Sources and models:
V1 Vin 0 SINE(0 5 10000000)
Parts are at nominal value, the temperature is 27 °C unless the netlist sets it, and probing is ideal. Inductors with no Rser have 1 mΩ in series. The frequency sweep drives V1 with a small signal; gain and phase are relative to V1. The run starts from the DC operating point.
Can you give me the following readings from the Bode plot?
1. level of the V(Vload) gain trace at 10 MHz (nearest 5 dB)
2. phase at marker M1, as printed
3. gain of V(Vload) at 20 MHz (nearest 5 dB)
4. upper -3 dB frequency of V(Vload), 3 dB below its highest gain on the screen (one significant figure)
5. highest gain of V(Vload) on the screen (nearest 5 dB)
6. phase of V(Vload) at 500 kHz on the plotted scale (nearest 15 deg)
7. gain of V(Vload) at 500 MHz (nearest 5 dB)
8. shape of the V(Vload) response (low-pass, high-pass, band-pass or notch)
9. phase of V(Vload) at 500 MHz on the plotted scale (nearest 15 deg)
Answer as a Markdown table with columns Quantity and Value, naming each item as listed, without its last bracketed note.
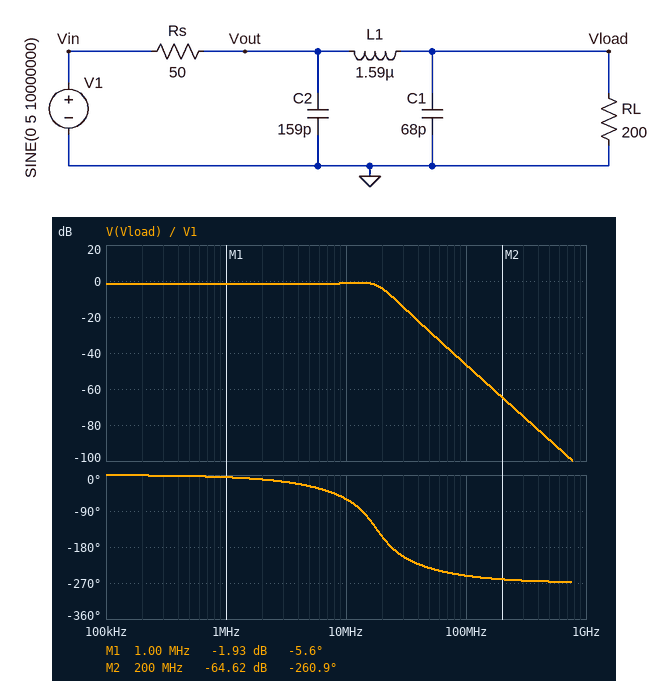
| Quantity | Value |
|---|---|
| level of the V(Vload) gain trace at 10 MHz | 0 dB |
| phase at marker M1, as printed | -5.6 deg |
| gain of V(Vload) at 20 MHz | -5 dB |
| upper -3 dB frequency of V(Vload), 3 dB below its highest gain on the screen | 20 MHz |
| highest gain of V(Vload) on the screen | 0 dB |
| phase of V(Vload) at 500 kHz on the plotted scale | 0 deg |
| gain of V(Vload) at 500 MHz | -90 dB |
| shape of the V(Vload) response | low-pass |
| phase of V(Vload) at 500 MHz on the plotted scale | -270 deg |
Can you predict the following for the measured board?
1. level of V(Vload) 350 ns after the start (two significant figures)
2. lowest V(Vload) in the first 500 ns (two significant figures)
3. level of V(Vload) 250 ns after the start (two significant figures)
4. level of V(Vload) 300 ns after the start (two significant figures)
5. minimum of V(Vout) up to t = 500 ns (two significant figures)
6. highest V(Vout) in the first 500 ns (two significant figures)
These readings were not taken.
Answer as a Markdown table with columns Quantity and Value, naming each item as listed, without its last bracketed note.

| Quantity | Value |
|---|---|
| level of V(Vload) 350 ns after the start | 3.8 V |
| lowest V(Vload) in the first 500 ns | -4.4 V |
| level of V(Vload) 250 ns after the start | 3.8 V |
| level of V(Vload) 300 ns after the start | -3.8 V |
| minimum of V(Vout) up to t = 500 ns | -3.3 V |
| highest V(Vout) in the first 500 ns | 3.6 V |
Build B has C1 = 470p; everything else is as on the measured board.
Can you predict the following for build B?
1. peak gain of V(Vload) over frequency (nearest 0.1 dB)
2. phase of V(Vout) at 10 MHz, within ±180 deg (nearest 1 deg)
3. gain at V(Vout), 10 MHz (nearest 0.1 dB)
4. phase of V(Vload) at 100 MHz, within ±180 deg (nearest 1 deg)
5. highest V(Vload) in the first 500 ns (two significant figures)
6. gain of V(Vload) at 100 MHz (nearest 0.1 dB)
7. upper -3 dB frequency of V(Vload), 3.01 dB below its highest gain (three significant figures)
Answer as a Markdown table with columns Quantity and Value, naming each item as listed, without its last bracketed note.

| Quantity | Value |
|---|---|
| peak gain of V(Vload) over frequency | -1.2 dB |
| phase of V(Vout) at 10 MHz, within ±180 deg | 13 deg |
| gain at V(Vout), 10 MHz | -0.7 dB |
| phase of V(Vload) at 100 MHz, within ±180 deg | 102 deg |
| highest V(Vload) in the first 500 ns | 2.6 V |
| gain of V(Vload) at 100 MHz | -63.4 dB |
| upper -3 dB frequency of V(Vload), 3.01 dB below its highest gain | 8.56 MHz |
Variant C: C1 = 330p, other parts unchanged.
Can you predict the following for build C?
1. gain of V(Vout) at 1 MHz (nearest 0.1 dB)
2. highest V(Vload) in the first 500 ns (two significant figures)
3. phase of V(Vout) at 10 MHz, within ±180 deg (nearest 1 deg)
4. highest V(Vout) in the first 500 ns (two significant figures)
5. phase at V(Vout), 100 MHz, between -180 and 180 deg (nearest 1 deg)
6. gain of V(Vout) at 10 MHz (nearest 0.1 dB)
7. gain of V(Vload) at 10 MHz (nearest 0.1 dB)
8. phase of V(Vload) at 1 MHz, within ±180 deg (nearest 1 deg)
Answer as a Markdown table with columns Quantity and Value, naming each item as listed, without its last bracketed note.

| Quantity | Value |
|---|---|
| gain of V(Vout) at 1 MHz | -2.1 dB |
| highest V(Vload) in the first 500 ns | 3.5 V |
| phase of V(Vout) at 10 MHz, within ±180 deg | 18 deg |
| highest V(Vout) in the first 500 ns | 4.0 V |
| phase at V(Vout), 100 MHz, between -180 and 180 deg | -79 deg |
| gain of V(Vout) at 10 MHz | -1.9 dB |
| gain of V(Vload) at 10 MHz | -3.3 dB |
| phase of V(Vload) at 1 MHz, within ±180 deg | -9 deg |
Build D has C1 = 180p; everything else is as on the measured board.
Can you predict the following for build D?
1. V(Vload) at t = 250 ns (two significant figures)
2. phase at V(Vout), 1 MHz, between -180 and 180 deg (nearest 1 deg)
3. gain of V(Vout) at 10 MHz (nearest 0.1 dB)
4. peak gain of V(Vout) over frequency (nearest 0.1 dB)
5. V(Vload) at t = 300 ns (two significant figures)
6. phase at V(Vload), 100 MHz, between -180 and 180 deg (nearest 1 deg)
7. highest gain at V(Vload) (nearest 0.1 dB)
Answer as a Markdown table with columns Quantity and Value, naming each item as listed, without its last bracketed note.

| Quantity | Value |
|---|---|
| V(Vload) at t = 250 ns | 4.9 V |
| phase at V(Vout), 1 MHz, between -180 and 180 deg | -4 deg |
| gain of V(Vout) at 10 MHz | -5.8 dB |
| peak gain of V(Vout) over frequency | -0.9 dB |
| V(Vload) at t = 300 ns | -4.9 V |
| phase at V(Vload), 100 MHz, between -180 and 180 deg | 104 deg |
| highest gain at V(Vload) | 0 dB |
